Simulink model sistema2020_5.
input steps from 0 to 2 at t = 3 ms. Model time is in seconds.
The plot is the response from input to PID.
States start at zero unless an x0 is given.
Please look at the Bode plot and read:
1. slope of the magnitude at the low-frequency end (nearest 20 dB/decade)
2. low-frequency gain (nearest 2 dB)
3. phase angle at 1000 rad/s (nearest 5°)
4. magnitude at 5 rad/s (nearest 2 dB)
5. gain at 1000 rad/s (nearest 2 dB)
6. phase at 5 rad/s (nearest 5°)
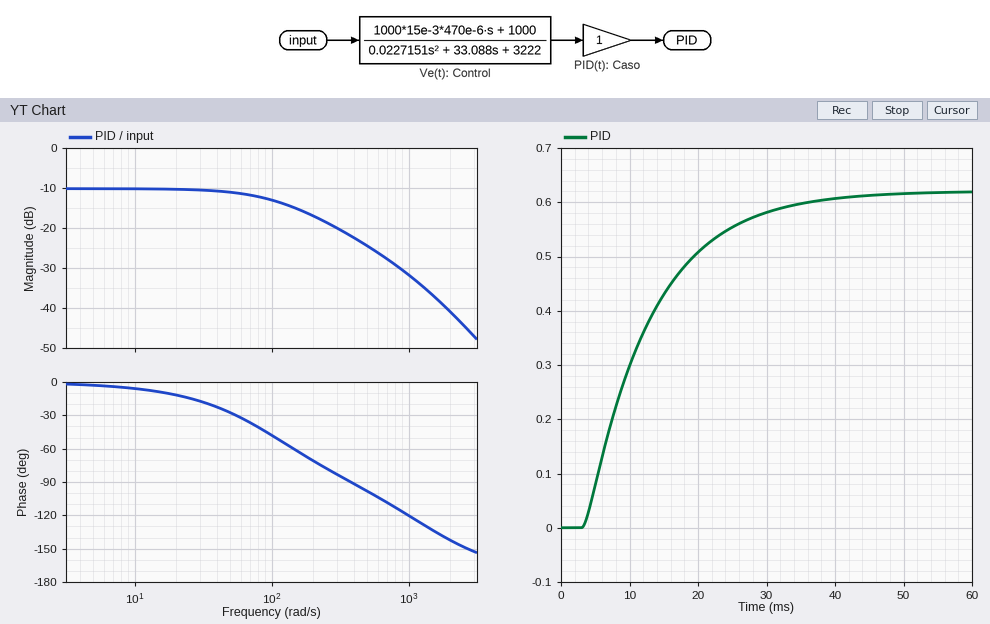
0 dB/decade
-10 dB
-120°
-10 dB
-32 dB
-5°
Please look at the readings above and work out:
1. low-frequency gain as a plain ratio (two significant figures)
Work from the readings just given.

0.32
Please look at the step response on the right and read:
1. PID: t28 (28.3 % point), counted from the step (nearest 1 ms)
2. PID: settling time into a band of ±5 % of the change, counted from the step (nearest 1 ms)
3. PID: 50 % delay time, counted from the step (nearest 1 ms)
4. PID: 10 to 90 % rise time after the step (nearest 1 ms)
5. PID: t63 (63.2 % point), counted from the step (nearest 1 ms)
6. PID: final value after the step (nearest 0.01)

4 ms
29 ms
7 ms
21 ms
10 ms
0.62
